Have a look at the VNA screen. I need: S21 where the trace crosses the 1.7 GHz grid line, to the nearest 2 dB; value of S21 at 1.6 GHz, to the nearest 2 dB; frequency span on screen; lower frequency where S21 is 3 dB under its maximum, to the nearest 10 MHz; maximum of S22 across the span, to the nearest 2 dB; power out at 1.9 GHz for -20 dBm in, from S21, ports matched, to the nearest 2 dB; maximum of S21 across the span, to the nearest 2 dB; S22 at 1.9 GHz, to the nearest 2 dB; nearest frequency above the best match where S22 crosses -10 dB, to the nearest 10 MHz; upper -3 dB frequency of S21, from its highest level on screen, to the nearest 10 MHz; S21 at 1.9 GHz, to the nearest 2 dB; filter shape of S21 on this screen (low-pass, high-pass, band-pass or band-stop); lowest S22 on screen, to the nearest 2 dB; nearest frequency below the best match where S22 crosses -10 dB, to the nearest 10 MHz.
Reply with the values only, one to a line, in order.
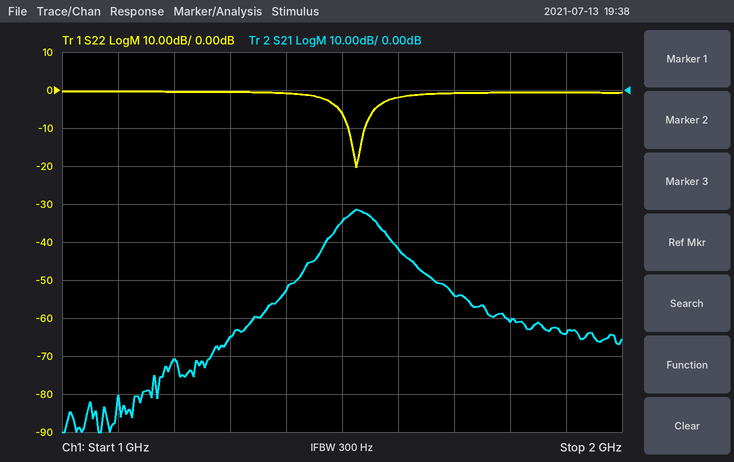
-54 dB
-42 dB
1 GHz
1.50 GHz
0 dB
-84 dBm
-32 dB
0 dB
1.54 GHz
1.56 GHz
-64 dB
band-pass
-20 dB
1.51 GHz
